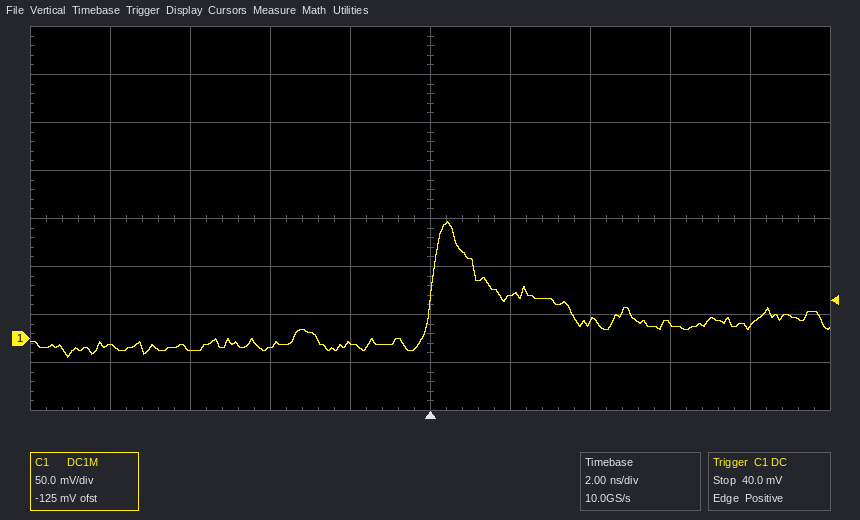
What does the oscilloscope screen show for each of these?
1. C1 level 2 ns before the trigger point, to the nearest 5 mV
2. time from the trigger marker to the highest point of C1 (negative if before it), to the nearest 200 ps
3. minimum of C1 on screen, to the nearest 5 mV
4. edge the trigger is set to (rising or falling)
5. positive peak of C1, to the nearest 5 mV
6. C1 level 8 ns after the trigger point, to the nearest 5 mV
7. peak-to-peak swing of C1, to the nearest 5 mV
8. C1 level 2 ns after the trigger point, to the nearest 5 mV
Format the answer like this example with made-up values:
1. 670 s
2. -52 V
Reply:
1. -5 mV
2. +400 ps
3. -20 mV
4. rising
5. 120 mV
6. 15 mV
7. 140 mV
8. 45 mV
